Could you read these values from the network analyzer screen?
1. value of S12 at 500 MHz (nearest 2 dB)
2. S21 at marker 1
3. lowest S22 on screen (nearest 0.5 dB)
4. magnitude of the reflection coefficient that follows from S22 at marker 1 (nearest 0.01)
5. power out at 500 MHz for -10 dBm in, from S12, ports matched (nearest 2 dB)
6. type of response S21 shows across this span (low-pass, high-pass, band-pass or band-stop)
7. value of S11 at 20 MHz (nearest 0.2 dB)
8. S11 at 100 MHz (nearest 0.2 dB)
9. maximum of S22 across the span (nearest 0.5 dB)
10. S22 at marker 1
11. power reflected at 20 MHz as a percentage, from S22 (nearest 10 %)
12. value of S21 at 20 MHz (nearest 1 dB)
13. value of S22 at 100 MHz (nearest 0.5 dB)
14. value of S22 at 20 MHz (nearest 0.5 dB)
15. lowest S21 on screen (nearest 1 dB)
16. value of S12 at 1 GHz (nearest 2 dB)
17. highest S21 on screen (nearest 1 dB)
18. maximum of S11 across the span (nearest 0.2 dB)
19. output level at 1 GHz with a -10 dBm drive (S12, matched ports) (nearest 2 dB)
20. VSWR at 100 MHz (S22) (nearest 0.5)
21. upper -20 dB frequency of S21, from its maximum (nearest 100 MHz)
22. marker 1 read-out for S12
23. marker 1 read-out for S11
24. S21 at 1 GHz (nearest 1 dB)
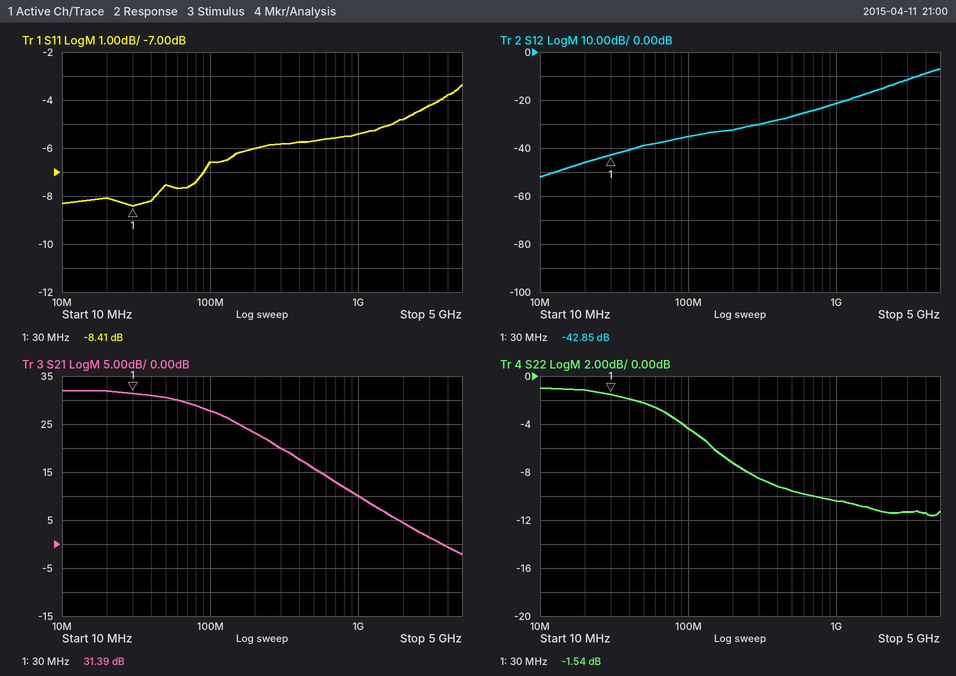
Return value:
-26 dB
31.39 dB
-11.5 dB
0.84
-36 dBm
low-pass
-8.0 dB
-6.6 dB
-1.0 dB
-1.54 dB
80 %
32 dB
-4.5 dB
-1.0 dB
-2 dB
-22 dB
32 dB
-3.4 dB
-32 dBm
4.0
800 MHz
-42.85 dB
-8.41 dB
10 dB
